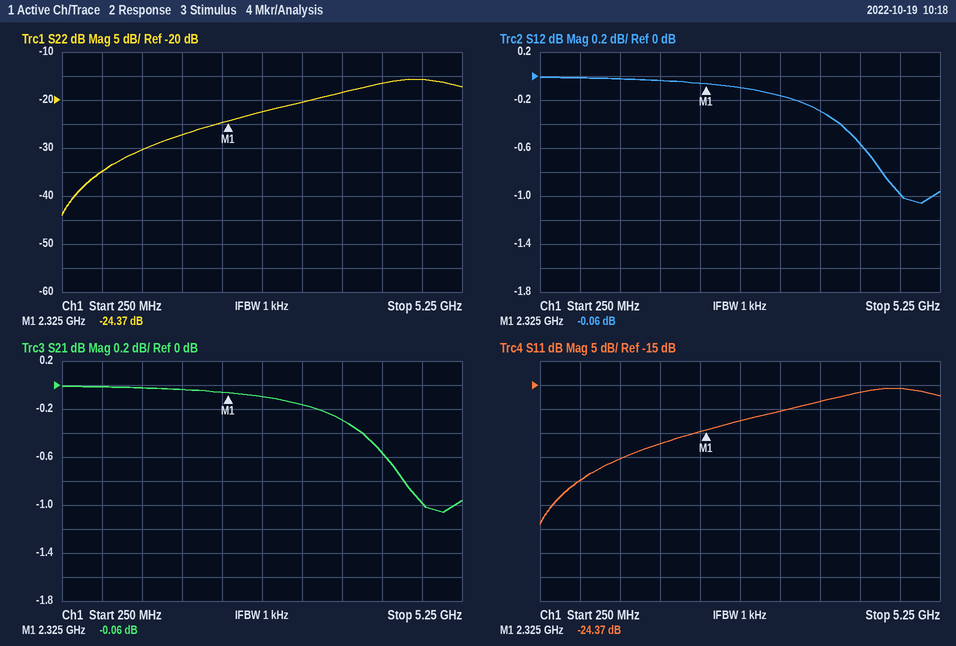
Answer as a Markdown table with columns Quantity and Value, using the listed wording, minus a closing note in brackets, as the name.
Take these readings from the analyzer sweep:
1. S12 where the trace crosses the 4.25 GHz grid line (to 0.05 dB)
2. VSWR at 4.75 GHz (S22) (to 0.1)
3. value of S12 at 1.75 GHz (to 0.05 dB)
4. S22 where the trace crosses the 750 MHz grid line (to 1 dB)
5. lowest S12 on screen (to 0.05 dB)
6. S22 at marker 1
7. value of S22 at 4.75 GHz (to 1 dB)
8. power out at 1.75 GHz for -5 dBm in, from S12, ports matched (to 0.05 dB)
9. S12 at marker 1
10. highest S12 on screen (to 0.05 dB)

| Quantity | Value |
|---|---|
| S12 where the trace crosses the 4.25 GHz grid line | -0.55 dB |
| VSWR at 4.75 GHz (S22) | 1.4 |
| value of S12 at 1.75 GHz | -0.05 dB |
| S22 where the trace crosses the 750 MHz grid line | -35 dB |
| lowest S12 on screen | -1.05 dB |
| S22 at marker 1 | -24.37 dB |
| value of S22 at 4.75 GHz | -16 dB |
| power out at 1.75 GHz for -5 dBm in, from S12, ports matched | -5.05 dBm |
| S12 at marker 1 | -0.06 dB |
| highest S12 on screen | 0.00 dB |
